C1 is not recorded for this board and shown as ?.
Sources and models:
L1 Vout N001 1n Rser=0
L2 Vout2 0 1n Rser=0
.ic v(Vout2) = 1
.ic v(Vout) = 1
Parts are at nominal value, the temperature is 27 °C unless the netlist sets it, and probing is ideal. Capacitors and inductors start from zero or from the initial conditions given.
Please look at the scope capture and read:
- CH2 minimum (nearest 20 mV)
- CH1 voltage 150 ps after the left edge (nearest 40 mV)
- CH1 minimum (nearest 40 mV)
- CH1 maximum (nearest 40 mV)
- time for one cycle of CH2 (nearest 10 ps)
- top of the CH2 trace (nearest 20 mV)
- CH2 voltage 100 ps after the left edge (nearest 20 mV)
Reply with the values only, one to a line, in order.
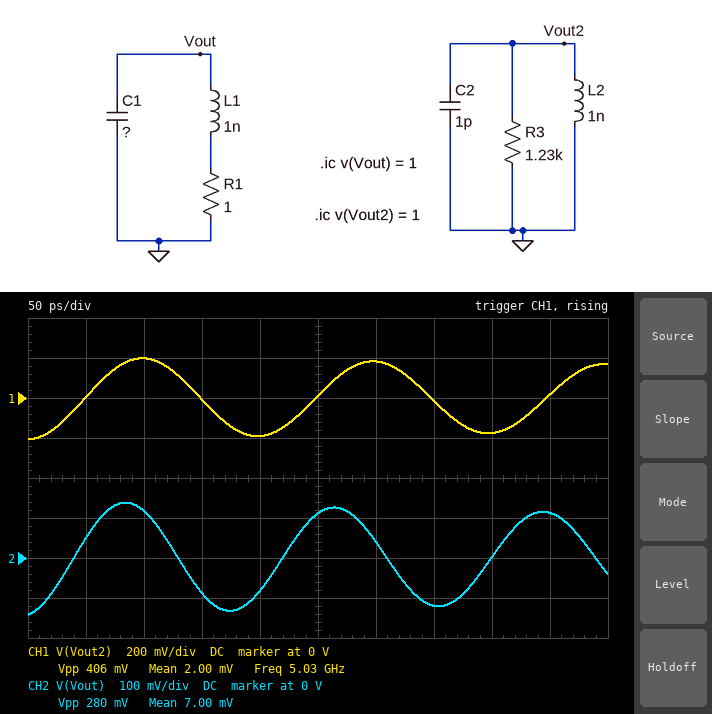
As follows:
-140 mV
0 V
-200 mV
200 mV
180 ps
140 mV
120 mV
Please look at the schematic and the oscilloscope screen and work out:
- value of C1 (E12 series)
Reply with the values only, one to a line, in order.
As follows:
820 fF
